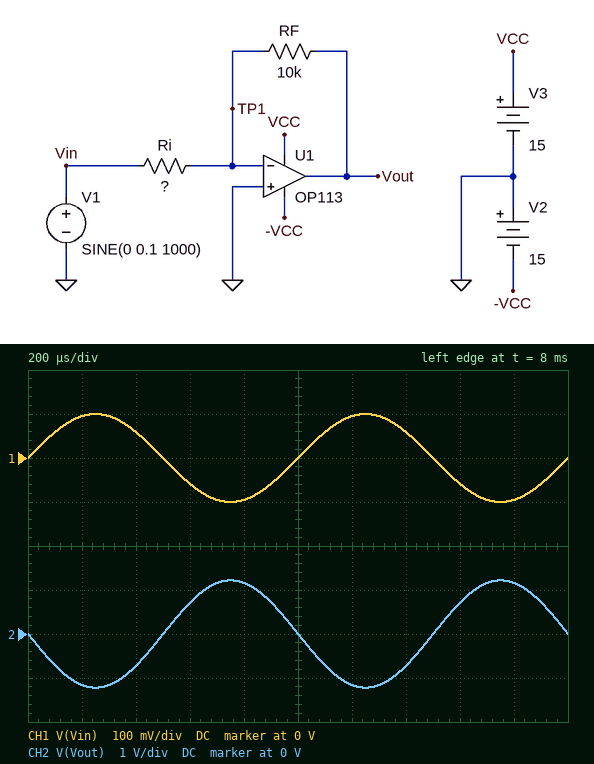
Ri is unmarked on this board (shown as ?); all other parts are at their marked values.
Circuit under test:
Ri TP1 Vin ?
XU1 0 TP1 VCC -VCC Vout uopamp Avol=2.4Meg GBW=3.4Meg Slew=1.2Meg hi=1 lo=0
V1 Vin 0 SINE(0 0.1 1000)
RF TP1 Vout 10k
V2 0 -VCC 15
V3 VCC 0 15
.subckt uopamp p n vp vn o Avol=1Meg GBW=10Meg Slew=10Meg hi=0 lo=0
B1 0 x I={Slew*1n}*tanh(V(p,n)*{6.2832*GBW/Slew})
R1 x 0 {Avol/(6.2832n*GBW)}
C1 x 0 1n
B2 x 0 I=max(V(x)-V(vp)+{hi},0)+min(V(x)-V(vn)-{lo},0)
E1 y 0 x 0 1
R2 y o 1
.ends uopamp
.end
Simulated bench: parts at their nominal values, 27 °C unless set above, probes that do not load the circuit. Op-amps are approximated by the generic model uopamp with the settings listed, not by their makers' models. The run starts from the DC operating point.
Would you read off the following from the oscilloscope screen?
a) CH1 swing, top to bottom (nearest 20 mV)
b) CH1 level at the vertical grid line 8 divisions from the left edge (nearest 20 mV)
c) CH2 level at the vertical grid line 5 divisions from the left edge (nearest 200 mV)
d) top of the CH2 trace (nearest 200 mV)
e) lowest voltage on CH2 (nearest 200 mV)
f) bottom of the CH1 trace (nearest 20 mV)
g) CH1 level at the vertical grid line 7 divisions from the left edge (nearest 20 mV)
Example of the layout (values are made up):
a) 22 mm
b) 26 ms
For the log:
a) 200 mV
b) -60 mV
c) 0 V
d) 1.2 V
e) -1.2 V
f) -100 mV
g) 60 mV
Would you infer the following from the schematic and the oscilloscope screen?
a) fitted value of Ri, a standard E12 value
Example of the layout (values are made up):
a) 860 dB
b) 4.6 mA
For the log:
a) 820 Ω
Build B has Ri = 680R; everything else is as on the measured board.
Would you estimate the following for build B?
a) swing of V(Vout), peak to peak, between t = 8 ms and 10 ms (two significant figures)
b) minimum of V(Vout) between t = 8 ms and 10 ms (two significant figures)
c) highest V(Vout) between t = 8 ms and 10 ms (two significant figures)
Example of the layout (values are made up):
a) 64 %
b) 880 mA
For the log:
a) 2.9 V
b) -1.5 V
c) 1.5 V
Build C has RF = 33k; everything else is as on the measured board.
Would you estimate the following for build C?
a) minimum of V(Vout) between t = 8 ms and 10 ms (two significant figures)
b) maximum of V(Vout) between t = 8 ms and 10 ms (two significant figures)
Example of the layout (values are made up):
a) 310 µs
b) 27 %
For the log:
a) -4.0 V
b) 4.0 V
